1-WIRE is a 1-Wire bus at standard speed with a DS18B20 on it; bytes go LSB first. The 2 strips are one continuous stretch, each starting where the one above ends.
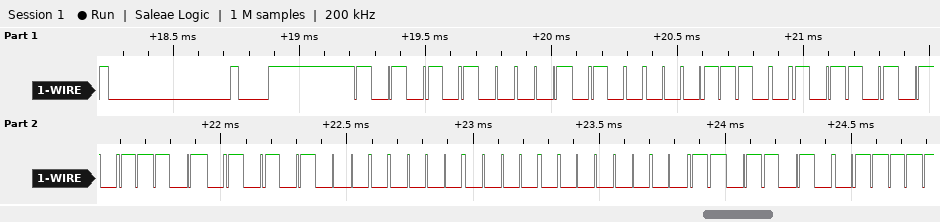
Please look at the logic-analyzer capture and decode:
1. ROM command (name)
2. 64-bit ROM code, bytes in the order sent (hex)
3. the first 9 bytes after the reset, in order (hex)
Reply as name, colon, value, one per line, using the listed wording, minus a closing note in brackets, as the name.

ROM command: Match ROM
64-bit ROM code, bytes in the order sent: 28 38 AD AE 0A 00 00 5B
the first 9 bytes after the reset, in order: 55 28 38 AD AE 0A 00 00 5B
